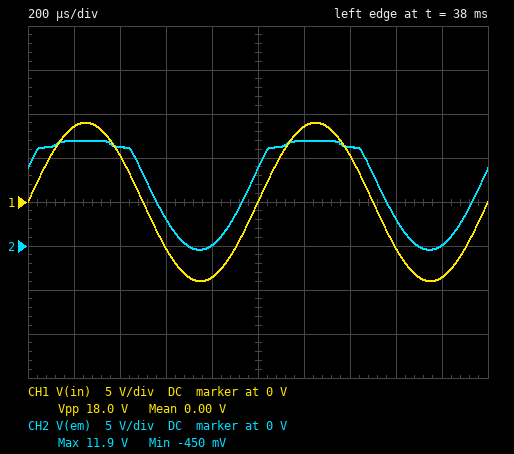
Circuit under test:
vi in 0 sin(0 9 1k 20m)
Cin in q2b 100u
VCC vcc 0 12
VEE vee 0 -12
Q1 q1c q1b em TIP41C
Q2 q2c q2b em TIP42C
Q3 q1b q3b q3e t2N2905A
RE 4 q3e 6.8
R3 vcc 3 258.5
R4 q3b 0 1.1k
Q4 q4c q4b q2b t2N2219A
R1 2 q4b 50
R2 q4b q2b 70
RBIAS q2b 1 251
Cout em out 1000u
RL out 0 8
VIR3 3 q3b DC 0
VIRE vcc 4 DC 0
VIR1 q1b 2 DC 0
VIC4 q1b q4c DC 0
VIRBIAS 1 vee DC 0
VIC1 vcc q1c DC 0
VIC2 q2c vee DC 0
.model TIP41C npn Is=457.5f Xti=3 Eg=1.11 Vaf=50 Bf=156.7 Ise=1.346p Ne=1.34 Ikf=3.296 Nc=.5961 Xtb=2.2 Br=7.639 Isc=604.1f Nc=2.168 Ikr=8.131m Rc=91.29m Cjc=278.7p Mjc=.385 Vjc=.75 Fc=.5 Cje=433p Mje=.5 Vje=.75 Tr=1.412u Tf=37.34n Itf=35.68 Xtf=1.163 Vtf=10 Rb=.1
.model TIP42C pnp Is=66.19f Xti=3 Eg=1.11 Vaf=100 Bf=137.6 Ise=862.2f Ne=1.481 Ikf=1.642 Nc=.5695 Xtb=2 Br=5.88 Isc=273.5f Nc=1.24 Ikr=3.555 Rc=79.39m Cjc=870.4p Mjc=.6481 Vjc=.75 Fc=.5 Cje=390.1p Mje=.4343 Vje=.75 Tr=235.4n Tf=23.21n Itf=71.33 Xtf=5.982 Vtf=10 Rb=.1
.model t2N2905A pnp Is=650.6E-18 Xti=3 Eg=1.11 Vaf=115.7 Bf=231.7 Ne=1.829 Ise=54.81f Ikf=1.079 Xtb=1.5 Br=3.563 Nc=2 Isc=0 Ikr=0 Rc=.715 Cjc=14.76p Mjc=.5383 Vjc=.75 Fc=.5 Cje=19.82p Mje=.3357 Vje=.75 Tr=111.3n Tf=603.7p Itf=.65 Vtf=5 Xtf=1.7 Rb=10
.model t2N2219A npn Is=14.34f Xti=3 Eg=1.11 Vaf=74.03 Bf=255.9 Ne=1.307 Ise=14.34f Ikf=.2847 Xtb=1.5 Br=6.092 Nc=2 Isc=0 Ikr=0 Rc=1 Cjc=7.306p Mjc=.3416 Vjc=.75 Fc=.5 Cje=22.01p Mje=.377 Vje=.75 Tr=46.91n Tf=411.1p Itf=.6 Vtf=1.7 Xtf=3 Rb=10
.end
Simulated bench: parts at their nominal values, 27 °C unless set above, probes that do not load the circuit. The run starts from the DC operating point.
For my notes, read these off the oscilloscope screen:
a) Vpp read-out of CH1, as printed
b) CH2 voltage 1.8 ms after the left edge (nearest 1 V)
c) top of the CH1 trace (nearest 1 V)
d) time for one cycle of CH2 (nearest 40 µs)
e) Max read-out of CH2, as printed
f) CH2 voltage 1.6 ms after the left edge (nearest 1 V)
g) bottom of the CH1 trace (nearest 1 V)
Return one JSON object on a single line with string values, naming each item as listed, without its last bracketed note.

{"Vpp read-out of CH1, as printed": "18.0 V", "CH2 voltage 1.8 ms after the left edge": "0 V", "top of the CH1 trace": "9 V", "time for one cycle of CH2": "1.00 ms", "Max read-out of CH2, as printed": "11.9 V", "CH2 voltage 1.6 ms after the left edge": "3 V", "bottom of the CH1 trace": "-9 V"}
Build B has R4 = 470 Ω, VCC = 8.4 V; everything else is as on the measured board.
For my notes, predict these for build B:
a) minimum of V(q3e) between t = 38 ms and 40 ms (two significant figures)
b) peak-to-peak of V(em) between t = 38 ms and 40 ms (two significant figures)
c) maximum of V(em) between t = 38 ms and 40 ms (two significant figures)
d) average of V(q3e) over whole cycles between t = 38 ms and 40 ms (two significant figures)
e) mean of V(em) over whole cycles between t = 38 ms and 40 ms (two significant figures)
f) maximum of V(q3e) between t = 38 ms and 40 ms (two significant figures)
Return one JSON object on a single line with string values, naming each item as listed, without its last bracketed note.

{"minimum of V(q3e) between t = 38 ms and 40 ms": "6.5 V", "peak-to-peak of V(em) between t = 38 ms and 40 ms": "10 V", "maximum of V(em) between t = 38 ms and 40 ms": "8.3 V", "average of V(q3e) over whole cycles between t = 38 ms and 40 ms": "7.6 V", "mean of V(em) over whole cycles between t = 38 ms and 40 ms": "4.6 V", "maximum of V(q3e) between t = 38 ms and 40 ms": "8.8 V"}
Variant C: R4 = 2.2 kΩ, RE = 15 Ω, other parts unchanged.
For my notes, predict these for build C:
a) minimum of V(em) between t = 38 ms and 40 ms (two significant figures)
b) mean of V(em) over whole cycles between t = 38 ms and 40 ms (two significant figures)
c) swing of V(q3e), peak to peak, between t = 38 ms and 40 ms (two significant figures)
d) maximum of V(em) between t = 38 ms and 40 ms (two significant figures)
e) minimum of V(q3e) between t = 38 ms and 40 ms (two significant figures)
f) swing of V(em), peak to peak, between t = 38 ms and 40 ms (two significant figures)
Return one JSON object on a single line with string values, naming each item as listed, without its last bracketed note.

{"minimum of V(em) between t = 38 ms and 40 ms": "-12 V", "mean of V(em) over whole cycles between t = 38 ms and 40 ms": "-3.1 V", "swing of V(q3e), peak to peak, between t = 38 ms and 40 ms": "6.7 mV", "maximum of V(em) between t = 38 ms and 40 ms": "5.7 V", "minimum of V(q3e) between t = 38 ms and 40 ms": "12 V", "swing of V(em), peak to peak, between t = 38 ms and 40 ms": "18 V"}
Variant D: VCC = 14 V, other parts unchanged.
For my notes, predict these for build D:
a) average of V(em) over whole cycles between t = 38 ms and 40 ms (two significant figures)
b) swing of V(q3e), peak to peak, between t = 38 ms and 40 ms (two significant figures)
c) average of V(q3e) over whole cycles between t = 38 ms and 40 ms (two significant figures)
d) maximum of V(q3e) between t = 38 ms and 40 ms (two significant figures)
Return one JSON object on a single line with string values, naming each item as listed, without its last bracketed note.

{"average of V(em) over whole cycles between t = 38 ms and 40 ms": "9.4 V", "swing of V(q3e), peak to peak, between t = 38 ms and 40 ms": "1.8 V", "average of V(q3e) over whole cycles between t = 38 ms and 40 ms": "13 V", "maximum of V(q3e) between t = 38 ms and 40 ms": "14 V"}
